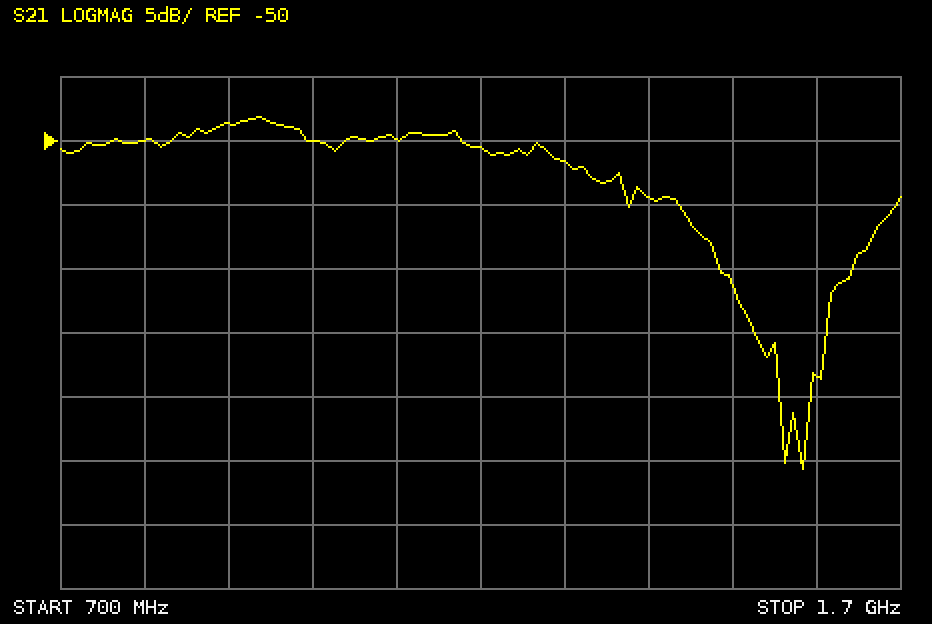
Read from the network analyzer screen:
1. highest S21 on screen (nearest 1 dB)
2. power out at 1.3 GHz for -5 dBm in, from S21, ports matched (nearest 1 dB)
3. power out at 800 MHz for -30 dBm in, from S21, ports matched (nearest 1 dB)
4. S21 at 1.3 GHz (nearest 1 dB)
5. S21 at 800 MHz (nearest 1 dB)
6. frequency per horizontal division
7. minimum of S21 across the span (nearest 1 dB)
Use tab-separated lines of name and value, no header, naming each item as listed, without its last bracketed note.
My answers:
highest S21 on screen	-48 dB
power out at 1.3 GHz for -5 dBm in, from S21, ports matched	-57 dBm
power out at 800 MHz for -30 dBm in, from S21, ports matched	-80 dBm
S21 at 1.3 GHz	-52 dB
S21 at 800 MHz	-50 dB
frequency per horizontal division	100 MHz
minimum of S21 across the span	-76 dB
